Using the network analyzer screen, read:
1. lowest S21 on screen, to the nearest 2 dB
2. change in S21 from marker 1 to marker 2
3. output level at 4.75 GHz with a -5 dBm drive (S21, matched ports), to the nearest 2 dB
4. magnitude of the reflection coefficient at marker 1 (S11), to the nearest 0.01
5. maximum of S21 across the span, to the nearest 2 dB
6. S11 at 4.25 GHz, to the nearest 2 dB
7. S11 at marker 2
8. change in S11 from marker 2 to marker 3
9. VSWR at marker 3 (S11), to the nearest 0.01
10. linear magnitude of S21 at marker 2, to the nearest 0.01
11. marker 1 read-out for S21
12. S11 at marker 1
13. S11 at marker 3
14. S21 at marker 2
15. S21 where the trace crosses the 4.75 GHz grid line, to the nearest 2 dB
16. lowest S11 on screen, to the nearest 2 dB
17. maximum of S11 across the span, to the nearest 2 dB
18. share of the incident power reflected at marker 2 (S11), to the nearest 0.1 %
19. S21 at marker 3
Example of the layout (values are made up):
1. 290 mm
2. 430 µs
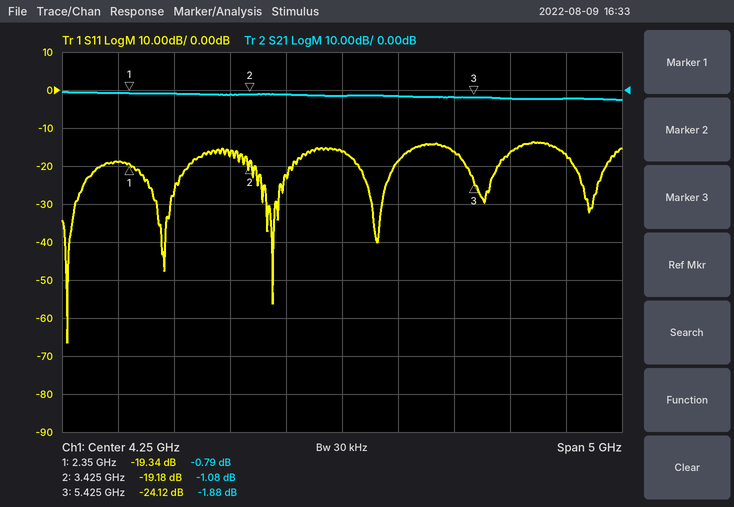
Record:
1. -2 dB
2. -0.29 dB
3. -6 dBm
4. 0.11
5. 0 dB
6. -16 dB
7. -19.18 dB
8. -4.94 dB
9. 1.13
10. 0.88
11. -0.79 dB
12. -19.34 dB
13. -24.12 dB
14. -1.08 dB
15. -2 dB
16. -66 dB
17. -14 dB
18. 1.2 %
19. -1.88 dB
